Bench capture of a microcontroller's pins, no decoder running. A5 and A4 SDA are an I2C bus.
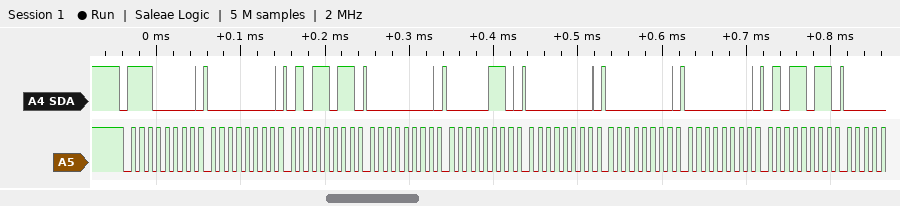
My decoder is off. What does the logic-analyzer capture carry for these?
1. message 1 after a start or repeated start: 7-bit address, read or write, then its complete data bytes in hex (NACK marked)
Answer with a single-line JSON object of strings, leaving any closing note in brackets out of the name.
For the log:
{"message 1 after a start or repeated start: 7-bit address, read or write, then its complete data bytes in hex": "0x70 write: 00 5B 00 06 00 00 00 5B"}
